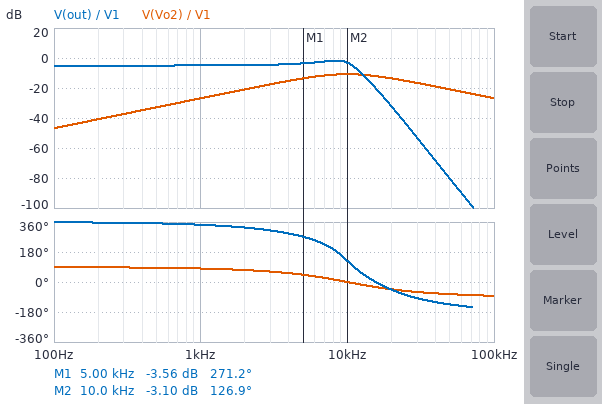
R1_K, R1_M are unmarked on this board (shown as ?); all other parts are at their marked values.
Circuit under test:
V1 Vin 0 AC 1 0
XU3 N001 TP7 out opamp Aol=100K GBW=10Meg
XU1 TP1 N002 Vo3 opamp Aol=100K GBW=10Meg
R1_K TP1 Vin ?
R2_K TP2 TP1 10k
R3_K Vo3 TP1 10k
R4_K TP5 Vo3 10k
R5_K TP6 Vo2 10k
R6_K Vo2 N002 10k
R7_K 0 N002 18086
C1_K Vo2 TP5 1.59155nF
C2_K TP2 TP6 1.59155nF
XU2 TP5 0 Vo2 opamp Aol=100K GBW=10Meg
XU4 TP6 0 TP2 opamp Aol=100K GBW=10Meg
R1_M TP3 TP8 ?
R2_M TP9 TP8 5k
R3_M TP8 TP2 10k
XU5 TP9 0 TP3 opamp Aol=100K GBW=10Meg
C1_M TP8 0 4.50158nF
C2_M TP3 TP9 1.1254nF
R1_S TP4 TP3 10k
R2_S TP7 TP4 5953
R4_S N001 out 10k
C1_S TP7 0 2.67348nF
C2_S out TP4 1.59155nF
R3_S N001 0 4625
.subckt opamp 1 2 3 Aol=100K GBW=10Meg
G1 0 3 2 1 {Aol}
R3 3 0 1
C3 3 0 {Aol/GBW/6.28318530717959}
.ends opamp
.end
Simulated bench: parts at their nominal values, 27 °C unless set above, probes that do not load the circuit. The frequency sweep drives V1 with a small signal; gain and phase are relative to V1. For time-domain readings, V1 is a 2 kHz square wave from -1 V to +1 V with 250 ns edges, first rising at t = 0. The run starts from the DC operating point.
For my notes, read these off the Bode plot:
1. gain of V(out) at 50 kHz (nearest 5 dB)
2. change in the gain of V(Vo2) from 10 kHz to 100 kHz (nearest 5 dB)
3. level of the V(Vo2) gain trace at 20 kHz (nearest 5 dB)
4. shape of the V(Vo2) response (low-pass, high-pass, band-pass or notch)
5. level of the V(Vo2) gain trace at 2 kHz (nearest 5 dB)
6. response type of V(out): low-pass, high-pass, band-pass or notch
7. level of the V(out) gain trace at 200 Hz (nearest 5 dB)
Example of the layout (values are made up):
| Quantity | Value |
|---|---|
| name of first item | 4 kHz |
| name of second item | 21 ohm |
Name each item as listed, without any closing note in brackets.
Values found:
| Quantity | Value |
|---|---|
| gain of V(out) at 50 kHz | -80 dB |
| change in the gain of V(Vo2) from 10 kHz to 100 kHz | -15 dB |
| level of the V(Vo2) gain trace at 20 kHz | -15 dB |
| shape of the V(Vo2) response | band-pass |
| level of the V(Vo2) gain trace at 2 kHz | -20 dB |
| response type of V(out): low-pass, high-pass, band-pass or notch | low-pass |
| level of the V(out) gain trace at 200 Hz | -5 dB |
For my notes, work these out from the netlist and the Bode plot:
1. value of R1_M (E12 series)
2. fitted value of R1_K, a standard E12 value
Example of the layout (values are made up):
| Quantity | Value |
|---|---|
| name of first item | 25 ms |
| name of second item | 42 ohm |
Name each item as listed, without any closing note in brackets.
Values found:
| Quantity | Value |
|---|---|
| value of R1_M | 3.9 kΩ |
| fitted value of R1_K, a standard E12 value | 22 kΩ |
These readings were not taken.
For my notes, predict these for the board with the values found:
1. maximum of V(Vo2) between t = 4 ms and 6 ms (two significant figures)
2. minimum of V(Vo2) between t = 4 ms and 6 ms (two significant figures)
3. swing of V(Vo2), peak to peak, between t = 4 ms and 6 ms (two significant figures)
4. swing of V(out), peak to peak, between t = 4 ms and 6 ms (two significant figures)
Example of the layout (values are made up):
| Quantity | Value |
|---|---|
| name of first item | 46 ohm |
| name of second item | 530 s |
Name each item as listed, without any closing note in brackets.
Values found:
| Quantity | Value |
|---|---|
| maximum of V(Vo2) between t = 4 ms and 6 ms | 390 mV |
| minimum of V(Vo2) between t = 4 ms and 6 ms | -390 mV |
| swing of V(Vo2), peak to peak, between t = 4 ms and 6 ms | 780 mV |
| swing of V(out), peak to peak, between t = 4 ms and 6 ms | 1.8 V |
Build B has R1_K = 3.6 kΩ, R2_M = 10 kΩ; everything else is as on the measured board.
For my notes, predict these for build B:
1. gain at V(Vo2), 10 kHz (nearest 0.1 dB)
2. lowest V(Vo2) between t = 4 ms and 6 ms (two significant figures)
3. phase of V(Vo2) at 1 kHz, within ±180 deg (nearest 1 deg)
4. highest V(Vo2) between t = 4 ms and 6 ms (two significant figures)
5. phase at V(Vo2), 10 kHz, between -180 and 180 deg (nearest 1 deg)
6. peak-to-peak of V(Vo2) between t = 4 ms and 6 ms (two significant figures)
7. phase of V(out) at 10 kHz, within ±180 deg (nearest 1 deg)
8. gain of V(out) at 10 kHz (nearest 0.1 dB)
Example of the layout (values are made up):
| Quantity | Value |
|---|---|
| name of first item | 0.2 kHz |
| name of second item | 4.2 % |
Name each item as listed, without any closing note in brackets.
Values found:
| Quantity | Value |
|---|---|
| gain at V(Vo2), 10 kHz | -0.9 dB |
| lowest V(Vo2) between t = 4 ms and 6 ms | -1.5 V |
| phase of V(Vo2) at 1 kHz, within ±180 deg | 73 deg |
| highest V(Vo2) between t = 4 ms and 6 ms | 1.5 V |
| phase at V(Vo2), 10 kHz, between -180 and 180 deg | 0 deg |
| peak-to-peak of V(Vo2) between t = 4 ms and 6 ms | 3.0 V |
| phase of V(out) at 10 kHz, within ±180 deg | 98 deg |
| gain of V(out) at 10 kHz | 4.5 dB |
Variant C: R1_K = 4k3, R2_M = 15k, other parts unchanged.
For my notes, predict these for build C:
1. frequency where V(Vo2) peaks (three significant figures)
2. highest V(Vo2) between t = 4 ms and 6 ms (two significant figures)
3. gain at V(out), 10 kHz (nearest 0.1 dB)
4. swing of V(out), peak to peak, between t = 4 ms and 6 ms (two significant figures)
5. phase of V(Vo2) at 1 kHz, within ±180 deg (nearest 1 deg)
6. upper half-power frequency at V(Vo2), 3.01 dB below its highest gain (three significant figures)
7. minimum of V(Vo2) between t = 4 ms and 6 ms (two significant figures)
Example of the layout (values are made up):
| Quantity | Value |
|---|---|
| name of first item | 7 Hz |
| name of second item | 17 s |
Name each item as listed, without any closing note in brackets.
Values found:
| Quantity | Value |
|---|---|
| frequency where V(Vo2) peaks | 10.1 kHz |
| highest V(Vo2) between t = 4 ms and 6 ms | 1.4 V |
| gain at V(out), 10 kHz | 1.1 dB |
| swing of V(out), peak to peak, between t = 4 ms and 6 ms | 5.8 V |
| phase of V(Vo2) at 1 kHz, within ±180 deg | 74 deg |
| upper half-power frequency at V(Vo2), 3.01 dB below its highest gain | 31.4 kHz |
| minimum of V(Vo2) between t = 4 ms and 6 ms | -1.4 V |
